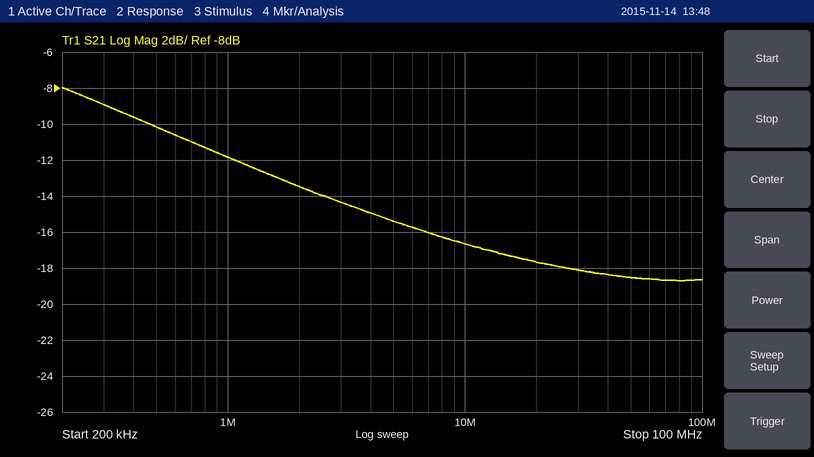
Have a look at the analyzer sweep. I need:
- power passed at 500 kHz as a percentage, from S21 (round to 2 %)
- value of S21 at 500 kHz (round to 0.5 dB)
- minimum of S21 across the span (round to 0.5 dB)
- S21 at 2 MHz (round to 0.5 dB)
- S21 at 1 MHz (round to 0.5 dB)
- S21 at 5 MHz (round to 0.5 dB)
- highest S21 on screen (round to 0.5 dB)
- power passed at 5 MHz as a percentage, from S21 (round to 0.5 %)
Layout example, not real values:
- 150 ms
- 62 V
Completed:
- 10 %
- -10.0 dB
- -18.5 dB
- -13.5 dB
- -12.0 dB
- -15.5 dB
- -8.0 dB
- 3.0 %
